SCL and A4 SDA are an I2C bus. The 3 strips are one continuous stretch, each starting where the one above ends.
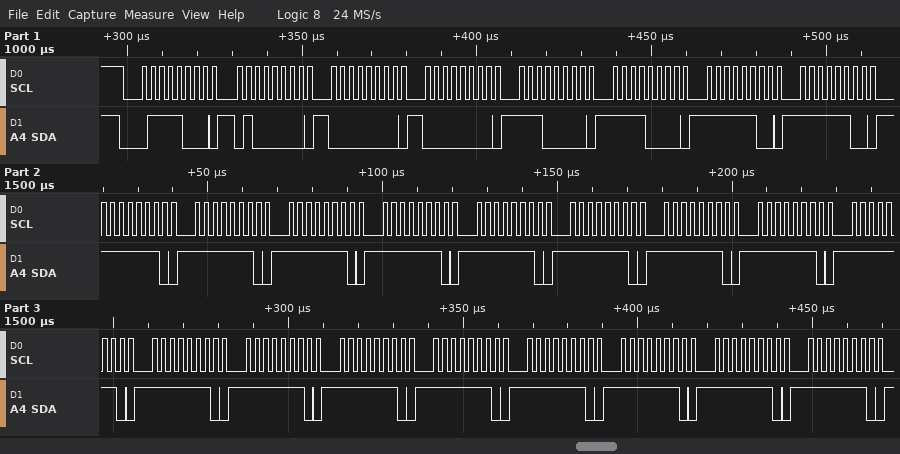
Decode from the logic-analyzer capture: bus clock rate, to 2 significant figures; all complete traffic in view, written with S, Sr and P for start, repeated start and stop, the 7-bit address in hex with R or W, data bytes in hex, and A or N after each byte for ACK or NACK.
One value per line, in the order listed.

400 kHz
S 3CW A 40 A 00 A 00 A E0 A F0 A FC A FC A FE A FE A FE A FE A FE A FE A FE A FE A FE A FE A FE A FE A FE A FE A FE A FE A FE A
